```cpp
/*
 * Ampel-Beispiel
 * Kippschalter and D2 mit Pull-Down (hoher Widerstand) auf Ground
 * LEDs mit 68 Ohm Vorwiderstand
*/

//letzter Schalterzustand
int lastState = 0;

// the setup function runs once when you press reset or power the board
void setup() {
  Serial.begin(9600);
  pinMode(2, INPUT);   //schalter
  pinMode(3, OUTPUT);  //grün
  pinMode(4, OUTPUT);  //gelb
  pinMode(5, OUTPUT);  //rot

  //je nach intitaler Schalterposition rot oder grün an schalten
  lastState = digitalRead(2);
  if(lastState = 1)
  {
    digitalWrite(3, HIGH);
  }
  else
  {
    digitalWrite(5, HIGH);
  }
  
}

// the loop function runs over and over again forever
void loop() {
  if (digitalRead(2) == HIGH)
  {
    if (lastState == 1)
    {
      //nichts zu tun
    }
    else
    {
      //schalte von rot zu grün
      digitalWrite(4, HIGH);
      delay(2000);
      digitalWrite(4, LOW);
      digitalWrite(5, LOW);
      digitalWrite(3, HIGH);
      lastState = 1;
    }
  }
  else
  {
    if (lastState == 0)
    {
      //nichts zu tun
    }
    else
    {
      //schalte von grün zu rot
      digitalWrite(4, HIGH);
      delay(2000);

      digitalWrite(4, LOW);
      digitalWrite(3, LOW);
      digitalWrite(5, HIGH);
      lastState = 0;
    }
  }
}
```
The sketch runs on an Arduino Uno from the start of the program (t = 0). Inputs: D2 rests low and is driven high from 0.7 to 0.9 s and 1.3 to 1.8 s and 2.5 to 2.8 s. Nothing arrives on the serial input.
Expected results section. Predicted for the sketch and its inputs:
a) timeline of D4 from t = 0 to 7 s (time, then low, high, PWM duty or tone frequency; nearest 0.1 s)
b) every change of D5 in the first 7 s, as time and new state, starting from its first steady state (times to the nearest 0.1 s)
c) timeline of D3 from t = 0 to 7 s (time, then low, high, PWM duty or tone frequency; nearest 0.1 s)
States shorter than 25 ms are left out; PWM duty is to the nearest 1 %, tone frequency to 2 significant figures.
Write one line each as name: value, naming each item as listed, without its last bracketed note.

timeline of D4 from t = 0 to 7 s: 0 s high; 2 s low; 2.5 s high; 6.5 s low
every change of D5 in the first 7 s, as time and new state, starting from its first steady state: 0 s low; 2 s high; 4.5 s low; 6.5 s high
timeline of D3 from t = 0 to 7 s: 0 s high; 2 s low; 4.5 s high; 6.5 s low
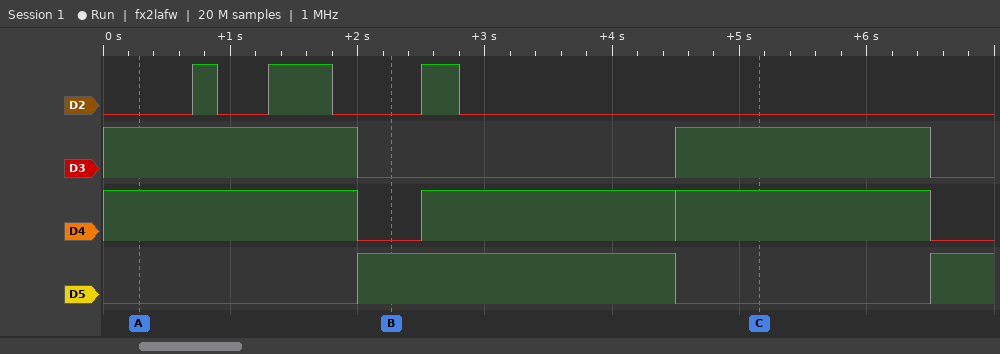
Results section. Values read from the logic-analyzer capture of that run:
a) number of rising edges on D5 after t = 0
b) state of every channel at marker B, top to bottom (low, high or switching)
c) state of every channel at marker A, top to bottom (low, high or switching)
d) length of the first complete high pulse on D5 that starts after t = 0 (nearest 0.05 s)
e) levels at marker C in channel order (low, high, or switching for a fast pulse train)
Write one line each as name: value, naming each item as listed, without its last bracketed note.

number of rising edges on D5 after t = 0: 2
state of every channel at marker B, top to bottom: D2 low, D3 low, D4 low, D5 high
state of every channel at marker A, top to bottom: D2 low, D3 high, D4 high, D5 low
length of the first complete high pulse on D5 that starts after t = 0: 2.50 s
levels at marker C in channel order: D2 low, D3 high, D4 high, D5 low
